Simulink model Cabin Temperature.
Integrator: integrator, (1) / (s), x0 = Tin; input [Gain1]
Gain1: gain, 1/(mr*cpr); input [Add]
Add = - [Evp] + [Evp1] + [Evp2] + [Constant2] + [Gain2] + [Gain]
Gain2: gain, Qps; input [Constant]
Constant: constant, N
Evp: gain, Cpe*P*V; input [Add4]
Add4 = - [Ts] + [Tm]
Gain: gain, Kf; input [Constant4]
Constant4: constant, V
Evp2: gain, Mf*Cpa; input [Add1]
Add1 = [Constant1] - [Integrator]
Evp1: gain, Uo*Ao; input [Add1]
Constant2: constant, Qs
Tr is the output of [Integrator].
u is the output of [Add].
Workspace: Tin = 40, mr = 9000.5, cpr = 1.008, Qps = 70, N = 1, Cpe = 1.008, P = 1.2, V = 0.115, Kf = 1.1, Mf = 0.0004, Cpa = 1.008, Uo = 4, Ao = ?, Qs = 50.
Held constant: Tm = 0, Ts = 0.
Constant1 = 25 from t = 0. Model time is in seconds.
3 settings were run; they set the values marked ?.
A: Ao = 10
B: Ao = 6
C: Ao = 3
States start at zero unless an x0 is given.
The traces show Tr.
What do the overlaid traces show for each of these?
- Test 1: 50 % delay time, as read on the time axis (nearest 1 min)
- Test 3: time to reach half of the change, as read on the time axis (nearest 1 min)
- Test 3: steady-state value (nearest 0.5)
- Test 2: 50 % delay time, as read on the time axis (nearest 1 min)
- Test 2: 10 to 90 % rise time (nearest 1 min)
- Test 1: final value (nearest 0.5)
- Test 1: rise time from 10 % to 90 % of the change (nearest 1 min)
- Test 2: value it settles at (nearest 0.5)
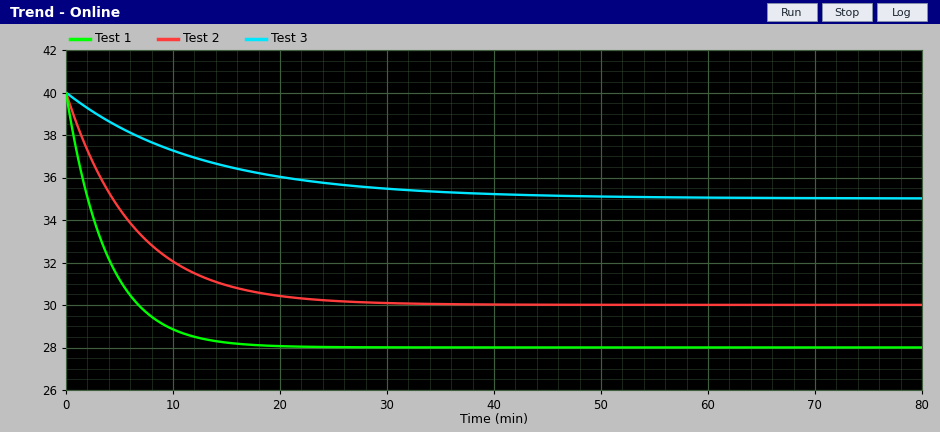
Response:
3 min
9 min
35.0
4 min
14 min
28.0
8 min
30.0
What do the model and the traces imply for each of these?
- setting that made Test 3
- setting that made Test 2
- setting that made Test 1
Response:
C
B
A
